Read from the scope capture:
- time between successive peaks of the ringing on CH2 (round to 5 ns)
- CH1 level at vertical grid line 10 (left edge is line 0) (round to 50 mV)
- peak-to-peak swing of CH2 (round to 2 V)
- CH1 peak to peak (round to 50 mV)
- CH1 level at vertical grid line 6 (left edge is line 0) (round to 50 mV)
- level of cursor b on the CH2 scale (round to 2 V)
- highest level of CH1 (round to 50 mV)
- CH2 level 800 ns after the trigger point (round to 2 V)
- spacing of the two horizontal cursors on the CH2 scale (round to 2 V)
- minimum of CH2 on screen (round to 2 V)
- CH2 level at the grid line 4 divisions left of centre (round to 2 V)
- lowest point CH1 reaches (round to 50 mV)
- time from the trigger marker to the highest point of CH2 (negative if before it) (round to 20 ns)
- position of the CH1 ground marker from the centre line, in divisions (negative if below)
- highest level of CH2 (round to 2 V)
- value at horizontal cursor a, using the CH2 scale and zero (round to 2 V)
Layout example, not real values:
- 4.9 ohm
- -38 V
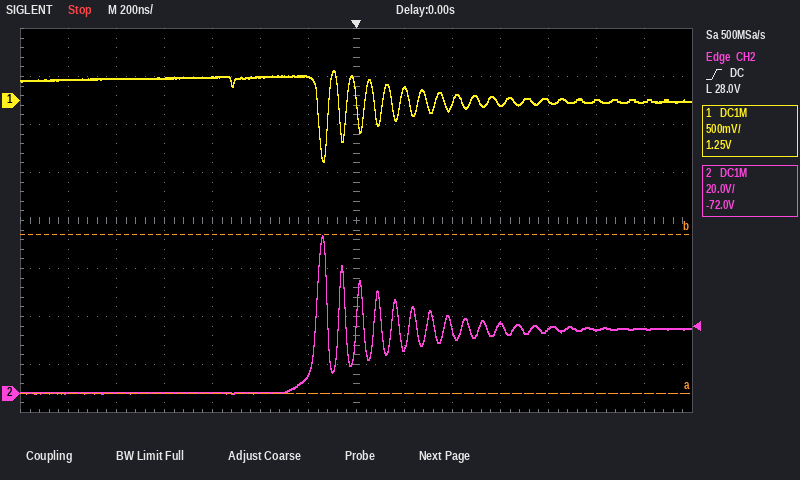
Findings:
- 75 ns
- -50 mV
- 66 V
- 950 mV
- 250 mV
- 66 V
- 300 mV
- 26 V
- 66 V
- 0 V
- 0 V
- -650 mV
- -140 ns
- +2.5 div
- 66 V
- 0 V
